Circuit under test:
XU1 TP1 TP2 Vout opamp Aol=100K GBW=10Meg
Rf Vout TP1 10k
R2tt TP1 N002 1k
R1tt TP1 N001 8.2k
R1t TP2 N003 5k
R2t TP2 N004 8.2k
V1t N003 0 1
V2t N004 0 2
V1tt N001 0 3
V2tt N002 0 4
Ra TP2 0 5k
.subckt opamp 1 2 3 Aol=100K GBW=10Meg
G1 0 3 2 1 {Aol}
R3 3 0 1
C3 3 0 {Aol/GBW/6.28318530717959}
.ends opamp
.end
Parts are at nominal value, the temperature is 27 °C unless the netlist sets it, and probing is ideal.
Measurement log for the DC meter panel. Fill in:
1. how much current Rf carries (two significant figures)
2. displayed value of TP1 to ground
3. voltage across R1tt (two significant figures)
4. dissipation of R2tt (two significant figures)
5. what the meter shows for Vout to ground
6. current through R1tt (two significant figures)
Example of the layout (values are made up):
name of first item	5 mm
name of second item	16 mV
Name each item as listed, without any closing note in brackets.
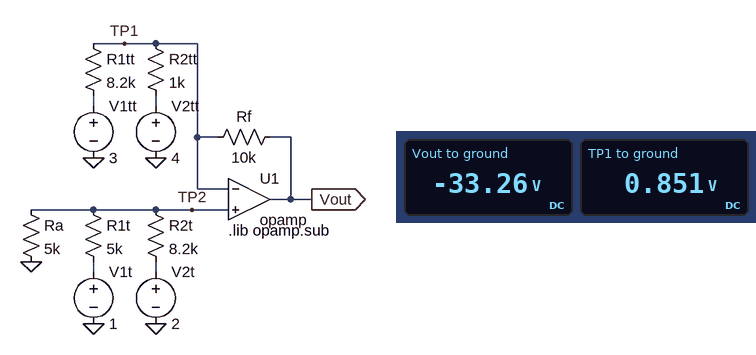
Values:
how much current Rf carries	3.4 mA
displayed value of TP1 to ground	0.851 V
voltage across R1tt	2.1 V
dissipation of R2tt	9.9 mW
what the meter shows for Vout to ground	-33.26 V
current through R1tt	260 µA
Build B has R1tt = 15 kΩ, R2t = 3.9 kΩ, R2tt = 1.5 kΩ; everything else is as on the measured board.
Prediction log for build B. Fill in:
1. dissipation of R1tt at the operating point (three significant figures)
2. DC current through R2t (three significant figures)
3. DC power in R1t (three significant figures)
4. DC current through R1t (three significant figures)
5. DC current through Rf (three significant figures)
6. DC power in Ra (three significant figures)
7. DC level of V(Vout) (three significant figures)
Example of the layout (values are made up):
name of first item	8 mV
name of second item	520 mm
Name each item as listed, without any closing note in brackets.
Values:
dissipation of R1tt at the operating point	244 µW
DC current through R2t	234 µA
DC power in R1t	1.48 µW
DC current through R1t	17.2 µA
DC current through Rf	2.07 mA
DC power in Ra	236 µW
DC level of V(Vout)	-19.6 V
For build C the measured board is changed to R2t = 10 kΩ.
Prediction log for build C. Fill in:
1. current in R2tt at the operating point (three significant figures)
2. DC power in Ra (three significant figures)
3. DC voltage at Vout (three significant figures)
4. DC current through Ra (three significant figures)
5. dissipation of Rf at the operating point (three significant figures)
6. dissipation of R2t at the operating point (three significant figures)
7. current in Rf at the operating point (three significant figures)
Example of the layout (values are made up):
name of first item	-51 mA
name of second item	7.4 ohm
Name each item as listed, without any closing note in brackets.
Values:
current in R2tt at the operating point	3.20 mA
DC power in Ra	128 µW
DC voltage at Vout	-33.9 V
DC current through Ra	160 µA
dissipation of Rf at the operating point	120 mW
dissipation of R2t at the operating point	144 µW
current in Rf at the operating point	3.47 mA
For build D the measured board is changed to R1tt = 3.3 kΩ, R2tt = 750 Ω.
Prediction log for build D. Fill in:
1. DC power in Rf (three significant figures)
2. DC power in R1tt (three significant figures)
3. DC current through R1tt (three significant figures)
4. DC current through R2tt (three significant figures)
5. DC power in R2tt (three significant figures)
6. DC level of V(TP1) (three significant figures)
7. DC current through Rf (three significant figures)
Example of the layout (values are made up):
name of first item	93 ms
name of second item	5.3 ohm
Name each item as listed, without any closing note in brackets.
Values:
DC power in Rf	235 mW
DC power in R1tt	1.40 mW
DC current through R1tt	651 µA
DC current through R2tt	4.20 mA
DC power in R2tt	13.2 mW
DC level of V(TP1)	851 mV
DC current through Rf	4.85 mA
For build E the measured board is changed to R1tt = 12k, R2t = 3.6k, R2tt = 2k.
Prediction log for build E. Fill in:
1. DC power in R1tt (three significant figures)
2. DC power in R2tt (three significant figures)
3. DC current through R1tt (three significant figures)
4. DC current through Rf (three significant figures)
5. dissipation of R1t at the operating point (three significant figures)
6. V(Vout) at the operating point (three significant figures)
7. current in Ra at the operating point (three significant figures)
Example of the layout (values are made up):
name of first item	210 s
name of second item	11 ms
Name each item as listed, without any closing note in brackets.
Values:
DC power in R1tt	296 µW
DC power in R2tt	4.16 mW
DC current through R1tt	157 µA
DC current through Rf	1.60 mA
dissipation of R1t at the operating point	2.63 µW
V(Vout) at the operating point	-14.9 V
current in Ra at the operating point	223 µA
